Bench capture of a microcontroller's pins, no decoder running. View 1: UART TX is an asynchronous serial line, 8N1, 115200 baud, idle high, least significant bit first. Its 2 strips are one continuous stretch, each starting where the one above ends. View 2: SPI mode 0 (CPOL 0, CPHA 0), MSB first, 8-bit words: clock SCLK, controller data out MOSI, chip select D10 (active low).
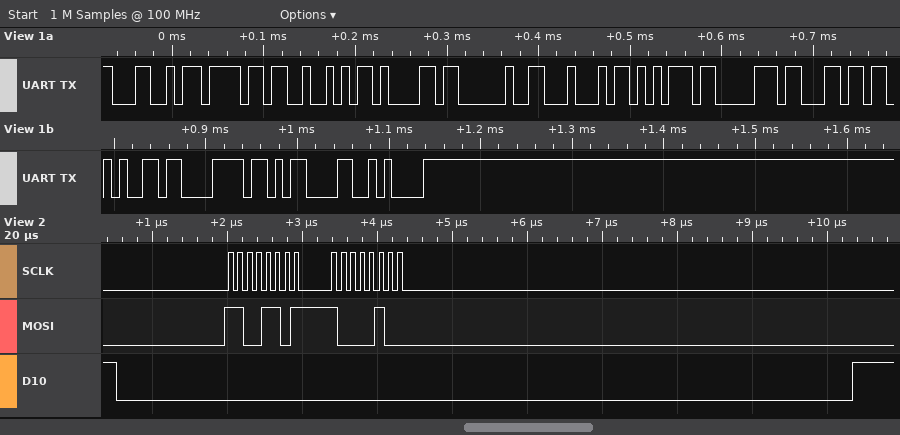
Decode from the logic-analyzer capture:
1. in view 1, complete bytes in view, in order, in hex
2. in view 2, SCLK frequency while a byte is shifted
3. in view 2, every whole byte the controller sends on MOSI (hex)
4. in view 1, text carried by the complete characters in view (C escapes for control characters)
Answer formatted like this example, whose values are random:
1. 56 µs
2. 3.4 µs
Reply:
1. 4C 6F 52 61 20 44 75 70 6C 65 78 0D 0A
2. 8 MHz
3. CD 84
4. "LoRa Duplex\r\n"
